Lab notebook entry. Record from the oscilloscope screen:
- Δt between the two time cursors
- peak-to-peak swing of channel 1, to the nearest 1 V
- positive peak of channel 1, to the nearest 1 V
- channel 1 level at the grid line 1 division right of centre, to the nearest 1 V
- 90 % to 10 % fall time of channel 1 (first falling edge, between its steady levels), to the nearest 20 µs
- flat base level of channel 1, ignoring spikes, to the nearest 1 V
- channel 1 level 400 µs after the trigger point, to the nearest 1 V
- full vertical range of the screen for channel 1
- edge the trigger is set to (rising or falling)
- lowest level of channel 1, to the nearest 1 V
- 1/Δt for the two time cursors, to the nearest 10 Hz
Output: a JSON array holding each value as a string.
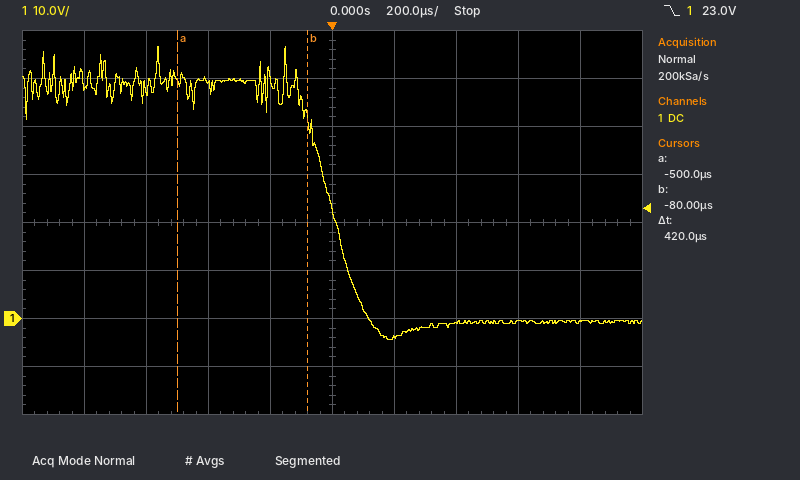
["420 µs", "61 V", "57 V", "-4 V", "180 µs", "-1 V", "-1 V", "80 V", "falling", "-4 V", "2.38 kHz"]
